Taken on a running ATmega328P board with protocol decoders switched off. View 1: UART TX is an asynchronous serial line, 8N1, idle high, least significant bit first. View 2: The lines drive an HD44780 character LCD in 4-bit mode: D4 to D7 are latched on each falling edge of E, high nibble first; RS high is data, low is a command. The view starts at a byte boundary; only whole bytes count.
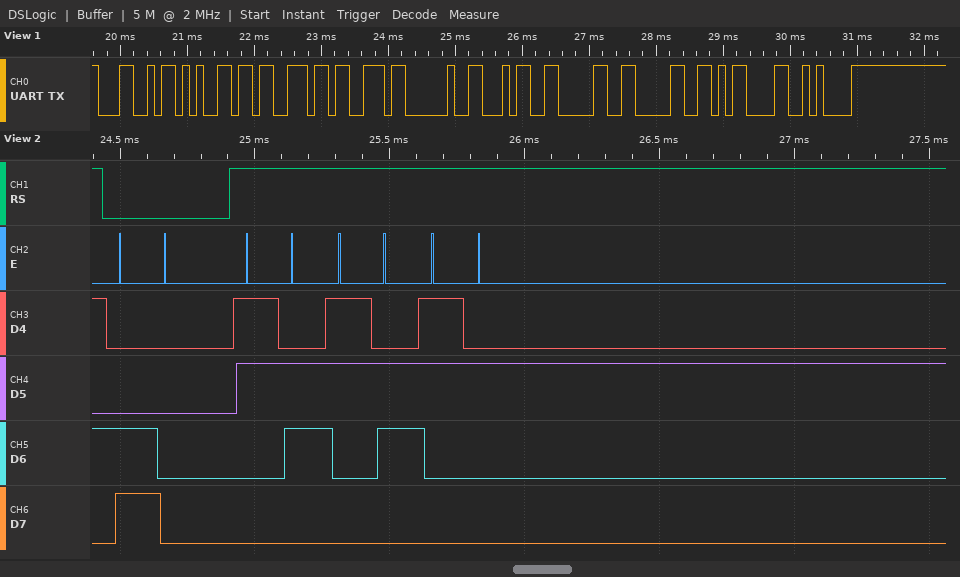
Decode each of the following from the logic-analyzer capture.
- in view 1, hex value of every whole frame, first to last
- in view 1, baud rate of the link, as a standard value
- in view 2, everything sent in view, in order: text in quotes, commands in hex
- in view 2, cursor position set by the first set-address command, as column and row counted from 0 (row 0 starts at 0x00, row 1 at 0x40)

0x4C 0x65 0x73 0x73 0x20 0x34 0x30 0x30 0x0D 0x0A
9600 baud
0xC0 "662"
column 0, row 1
